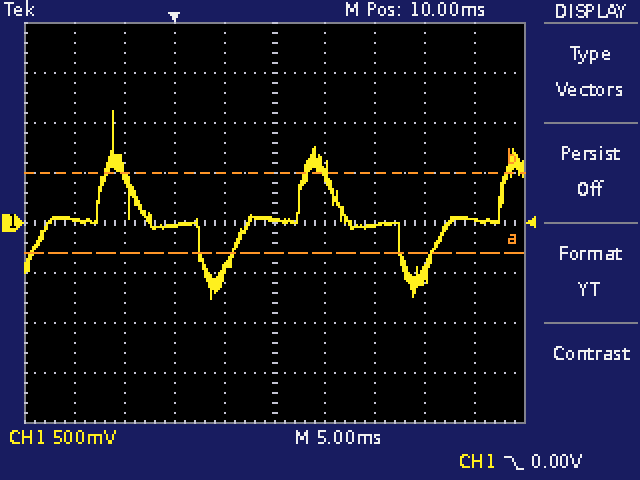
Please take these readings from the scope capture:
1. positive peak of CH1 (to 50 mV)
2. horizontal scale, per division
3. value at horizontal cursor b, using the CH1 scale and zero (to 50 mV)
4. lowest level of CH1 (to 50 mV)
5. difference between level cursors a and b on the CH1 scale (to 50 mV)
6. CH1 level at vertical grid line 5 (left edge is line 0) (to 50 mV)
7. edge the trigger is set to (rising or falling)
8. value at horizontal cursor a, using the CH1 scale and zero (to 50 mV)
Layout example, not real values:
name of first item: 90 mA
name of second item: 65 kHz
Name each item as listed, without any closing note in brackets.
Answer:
positive peak of CH1: 1.10 V
horizontal scale, per division: 5 ms
value at horizontal cursor b, using the CH1 scale and zero: 500 mV
lowest level of CH1: -750 mV
difference between level cursors a and b on the CH1 scale: 800 mV
CH1 level at vertical grid line 5 (left edge is line 0): 50 mV
edge the trigger is set to: falling
value at horizontal cursor a, using the CH1 scale and zero: -300 mV
